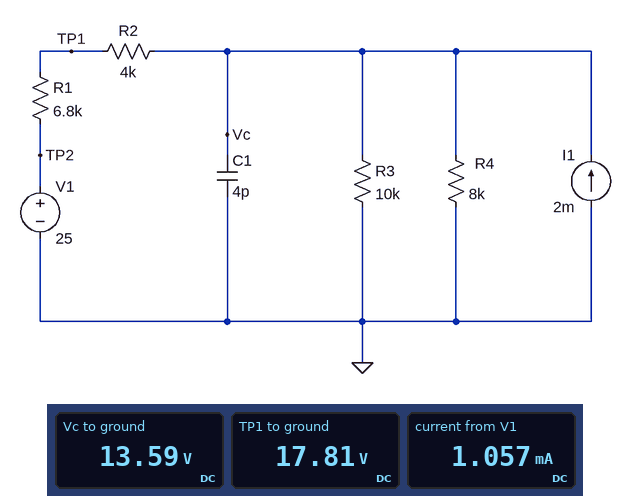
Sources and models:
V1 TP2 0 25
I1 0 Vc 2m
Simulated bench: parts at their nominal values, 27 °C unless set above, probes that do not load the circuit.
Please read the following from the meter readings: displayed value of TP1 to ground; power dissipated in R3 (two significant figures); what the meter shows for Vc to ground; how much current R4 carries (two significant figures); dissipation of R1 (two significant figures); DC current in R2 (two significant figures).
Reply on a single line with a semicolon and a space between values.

17.81 V; 18 mW; 13.59 V; 1.7 mA; 7.6 mW; 1.1 mA
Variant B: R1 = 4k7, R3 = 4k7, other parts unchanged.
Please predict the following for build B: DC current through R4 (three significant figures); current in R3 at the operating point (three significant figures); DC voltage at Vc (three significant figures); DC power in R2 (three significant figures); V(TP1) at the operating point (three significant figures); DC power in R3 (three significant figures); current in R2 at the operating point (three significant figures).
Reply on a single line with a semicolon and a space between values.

1.35 mA; 2.29 mA; 10.8 V; 10.7 mW; 17.3 V; 24.7 mW; 1.64 mA
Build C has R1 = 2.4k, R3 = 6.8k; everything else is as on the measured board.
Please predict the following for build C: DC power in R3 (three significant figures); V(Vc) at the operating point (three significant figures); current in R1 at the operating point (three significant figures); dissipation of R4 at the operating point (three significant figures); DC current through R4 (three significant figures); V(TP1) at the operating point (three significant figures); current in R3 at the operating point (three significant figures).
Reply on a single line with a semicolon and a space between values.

28.0 mW; 13.8 V; 1.75 mA; 23.8 mW; 1.72 mA; 20.8 V; 2.03 mA
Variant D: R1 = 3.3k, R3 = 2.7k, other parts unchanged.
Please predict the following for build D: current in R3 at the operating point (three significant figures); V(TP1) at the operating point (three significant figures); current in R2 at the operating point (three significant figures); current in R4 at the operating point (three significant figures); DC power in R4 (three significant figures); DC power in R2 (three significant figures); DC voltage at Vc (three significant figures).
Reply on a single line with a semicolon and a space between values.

3.18 mA; 17.6 V; 2.25 mA; 1.07 mA; 9.20 mW; 20.2 mW; 8.58 V
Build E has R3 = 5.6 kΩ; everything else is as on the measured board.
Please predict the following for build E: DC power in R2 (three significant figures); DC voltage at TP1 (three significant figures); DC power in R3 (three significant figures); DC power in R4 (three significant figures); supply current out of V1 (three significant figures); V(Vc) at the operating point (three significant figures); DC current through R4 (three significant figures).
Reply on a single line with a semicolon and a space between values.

6.83 mW; 16.1 V; 21.2 mW; 14.8 mW; 1.31 mA; 10.9 V; 1.36 mA
